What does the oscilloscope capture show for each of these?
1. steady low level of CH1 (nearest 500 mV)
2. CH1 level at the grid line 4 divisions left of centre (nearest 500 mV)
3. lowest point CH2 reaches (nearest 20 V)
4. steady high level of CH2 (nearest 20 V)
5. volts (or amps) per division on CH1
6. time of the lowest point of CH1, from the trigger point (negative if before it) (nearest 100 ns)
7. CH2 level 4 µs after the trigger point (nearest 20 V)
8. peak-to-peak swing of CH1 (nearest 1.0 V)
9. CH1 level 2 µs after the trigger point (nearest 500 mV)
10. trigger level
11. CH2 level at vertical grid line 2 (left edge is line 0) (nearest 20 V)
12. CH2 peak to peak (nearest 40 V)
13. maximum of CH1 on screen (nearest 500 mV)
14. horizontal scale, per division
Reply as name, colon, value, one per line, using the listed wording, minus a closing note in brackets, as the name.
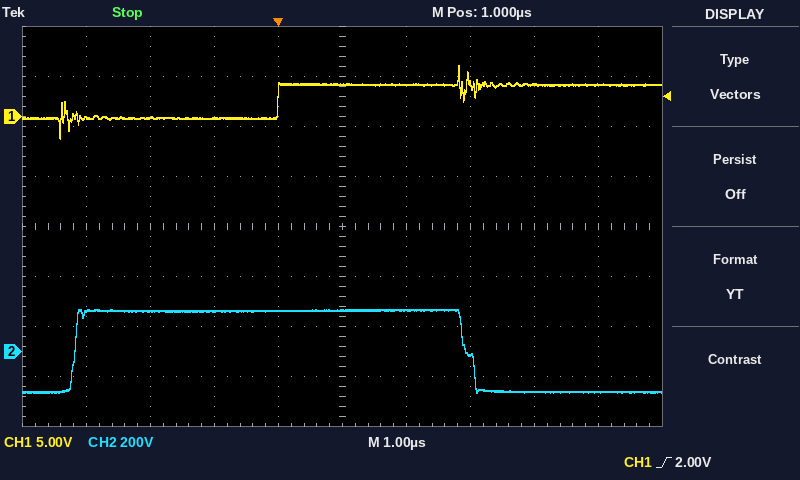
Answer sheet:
steady low level of CH1: 0.0 V
CH1 level at the grid line 4 divisions left of centre: 0.0 V
lowest point CH2 reaches: -160 V
steady high level of CH2: 160 V
volts (or amps) per division on CH1: 5 V
time of the lowest point of CH1, from the trigger point (negative if before it): -3.4 µs
CH2 level 4 µs after the trigger point: -160 V
peak-to-peak swing of CH1: 7.0 V
CH1 level 2 µs after the trigger point: 3.0 V
trigger level: 2.00 V
CH2 level at vertical grid line 2 (left edge is line 0): 160 V
CH2 peak to peak: 320 V
maximum of CH1 on screen: 5.0 V
horizontal scale, per division: 1 µs
